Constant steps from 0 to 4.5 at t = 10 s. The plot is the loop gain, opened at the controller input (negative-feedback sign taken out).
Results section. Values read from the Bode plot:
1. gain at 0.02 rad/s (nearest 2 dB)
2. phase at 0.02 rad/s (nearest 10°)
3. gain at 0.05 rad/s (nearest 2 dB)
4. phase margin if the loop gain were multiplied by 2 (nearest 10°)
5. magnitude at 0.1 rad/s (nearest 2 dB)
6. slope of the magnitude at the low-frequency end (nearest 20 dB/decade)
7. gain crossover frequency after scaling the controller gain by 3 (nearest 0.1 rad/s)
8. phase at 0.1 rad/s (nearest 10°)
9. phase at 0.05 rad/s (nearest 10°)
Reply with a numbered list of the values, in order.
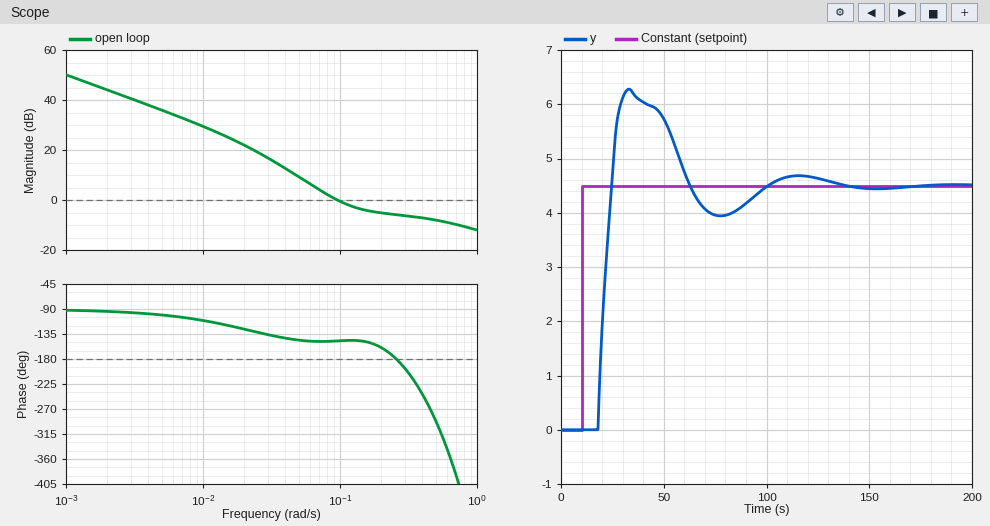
1. 22 dB
2. -130°
3. 10 dB
4. -10°
5. 0 dB
6. -20 dB/decade
7. 0.7 rad/s
8. -150°
9. -150°
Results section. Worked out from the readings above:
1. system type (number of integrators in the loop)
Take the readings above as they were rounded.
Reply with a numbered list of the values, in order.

1. 1
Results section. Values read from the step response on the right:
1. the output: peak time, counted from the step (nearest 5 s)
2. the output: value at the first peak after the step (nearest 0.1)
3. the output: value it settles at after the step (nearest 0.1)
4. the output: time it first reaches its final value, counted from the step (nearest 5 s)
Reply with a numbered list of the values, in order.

1. 25 s
2. 6.3
3. 4.5
4. 15 s
